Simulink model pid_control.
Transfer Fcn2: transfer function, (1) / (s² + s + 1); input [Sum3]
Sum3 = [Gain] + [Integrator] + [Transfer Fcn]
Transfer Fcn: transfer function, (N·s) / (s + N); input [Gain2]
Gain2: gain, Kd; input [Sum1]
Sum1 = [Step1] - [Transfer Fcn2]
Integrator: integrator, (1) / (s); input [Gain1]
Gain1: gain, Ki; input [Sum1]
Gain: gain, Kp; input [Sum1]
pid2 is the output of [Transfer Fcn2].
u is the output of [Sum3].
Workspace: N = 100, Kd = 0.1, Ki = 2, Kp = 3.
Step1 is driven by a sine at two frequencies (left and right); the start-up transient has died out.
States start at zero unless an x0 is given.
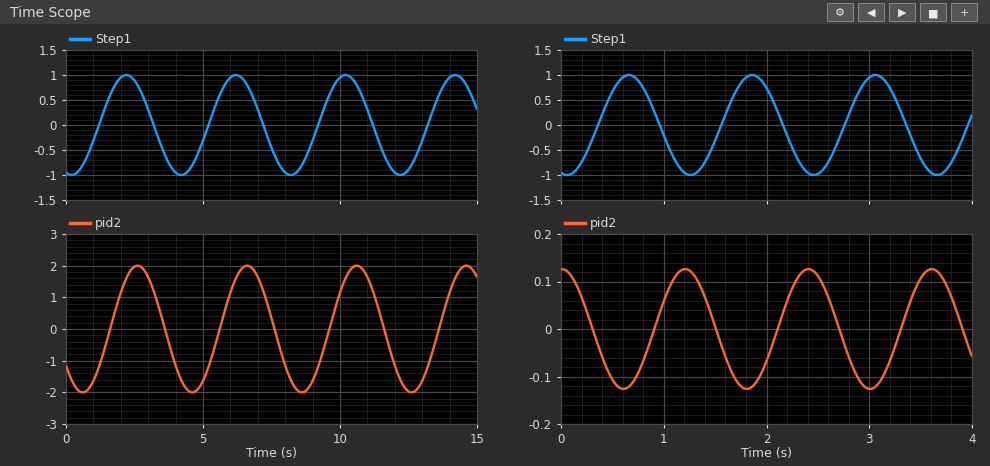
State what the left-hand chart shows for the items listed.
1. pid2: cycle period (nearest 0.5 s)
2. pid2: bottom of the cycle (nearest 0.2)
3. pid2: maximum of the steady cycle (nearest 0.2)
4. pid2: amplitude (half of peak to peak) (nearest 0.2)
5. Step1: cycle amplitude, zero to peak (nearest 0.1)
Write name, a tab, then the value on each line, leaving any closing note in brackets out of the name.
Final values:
pid2: cycle period	4.0 s
pid2: bottom of the cycle	-2.0
pid2: maximum of the steady cycle	2.0
pid2: amplitude (half of peak to peak)	2.0
Step1: cycle amplitude, zero to peak	1.0
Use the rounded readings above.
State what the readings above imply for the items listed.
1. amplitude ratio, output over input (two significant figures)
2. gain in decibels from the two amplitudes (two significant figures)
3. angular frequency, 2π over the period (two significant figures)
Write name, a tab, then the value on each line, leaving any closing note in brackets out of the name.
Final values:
amplitude ratio, output over input	2.0
gain in decibels from the two amplitudes	6.0 dB
angular frequency, 2π over the period	1.6 rad/s
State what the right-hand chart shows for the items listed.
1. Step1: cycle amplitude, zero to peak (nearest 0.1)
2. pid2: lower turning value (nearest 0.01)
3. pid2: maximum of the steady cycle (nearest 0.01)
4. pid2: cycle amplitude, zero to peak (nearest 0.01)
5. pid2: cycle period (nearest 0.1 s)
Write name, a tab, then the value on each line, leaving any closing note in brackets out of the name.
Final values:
Step1: cycle amplitude, zero to peak	1.0
pid2: lower turning value	-0.13
pid2: maximum of the steady cycle	0.13
pid2: cycle amplitude, zero to peak	0.13
pid2: cycle period	1.2 s
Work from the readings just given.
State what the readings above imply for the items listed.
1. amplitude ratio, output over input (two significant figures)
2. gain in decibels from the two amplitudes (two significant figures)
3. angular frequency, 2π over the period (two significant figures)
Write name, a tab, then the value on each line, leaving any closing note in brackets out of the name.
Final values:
amplitude ratio, output over input	0.13
gain in decibels from the two amplitudes	-18 dB
angular frequency, 2π over the period	5.2 rad/s
